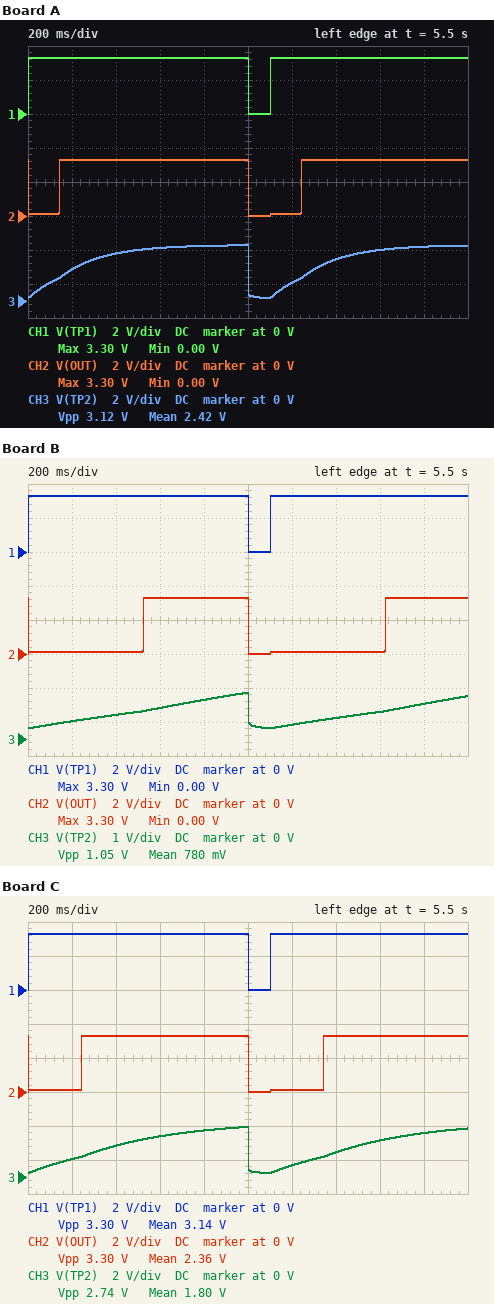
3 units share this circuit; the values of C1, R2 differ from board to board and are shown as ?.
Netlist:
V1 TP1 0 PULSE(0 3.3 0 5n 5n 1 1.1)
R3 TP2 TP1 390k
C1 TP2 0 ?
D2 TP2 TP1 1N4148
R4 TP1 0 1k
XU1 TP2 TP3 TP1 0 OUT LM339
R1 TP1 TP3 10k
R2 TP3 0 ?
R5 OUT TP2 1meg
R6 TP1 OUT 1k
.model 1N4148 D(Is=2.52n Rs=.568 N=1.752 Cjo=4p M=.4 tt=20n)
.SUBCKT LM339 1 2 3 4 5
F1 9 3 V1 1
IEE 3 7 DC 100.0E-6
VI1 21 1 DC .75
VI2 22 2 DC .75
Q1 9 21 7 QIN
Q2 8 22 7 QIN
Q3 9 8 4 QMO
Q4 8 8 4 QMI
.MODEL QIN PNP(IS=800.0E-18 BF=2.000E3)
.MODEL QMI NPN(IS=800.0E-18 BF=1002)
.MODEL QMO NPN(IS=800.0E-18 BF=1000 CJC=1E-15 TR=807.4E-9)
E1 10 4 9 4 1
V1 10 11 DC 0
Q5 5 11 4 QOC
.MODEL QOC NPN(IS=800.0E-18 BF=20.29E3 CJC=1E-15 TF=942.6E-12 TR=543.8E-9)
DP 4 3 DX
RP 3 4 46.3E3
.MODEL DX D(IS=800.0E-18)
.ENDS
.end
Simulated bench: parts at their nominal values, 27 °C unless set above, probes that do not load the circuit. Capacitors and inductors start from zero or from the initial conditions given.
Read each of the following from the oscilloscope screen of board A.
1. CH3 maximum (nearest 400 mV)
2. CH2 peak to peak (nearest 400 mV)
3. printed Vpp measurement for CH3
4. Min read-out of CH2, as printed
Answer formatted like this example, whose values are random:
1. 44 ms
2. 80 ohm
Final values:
1. 3.2 V
2. 3.2 V
3. 3.12 V
4. 0.00 V
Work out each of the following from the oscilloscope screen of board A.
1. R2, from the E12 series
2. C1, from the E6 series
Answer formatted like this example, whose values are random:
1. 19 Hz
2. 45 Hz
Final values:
1. 6.8 kΩ
2. 680 nF
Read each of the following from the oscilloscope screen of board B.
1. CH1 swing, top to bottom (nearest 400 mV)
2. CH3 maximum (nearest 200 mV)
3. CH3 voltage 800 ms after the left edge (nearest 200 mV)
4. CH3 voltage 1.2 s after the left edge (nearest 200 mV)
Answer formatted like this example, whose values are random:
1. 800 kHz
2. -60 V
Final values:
1. 3.2 V
2. 1.4 V
3. 1.2 V
4. 400 mV
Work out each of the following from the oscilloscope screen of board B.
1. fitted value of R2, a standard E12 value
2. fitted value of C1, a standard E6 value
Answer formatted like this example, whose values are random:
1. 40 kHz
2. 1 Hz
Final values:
1. 3.3 kΩ
2. 6.8 µF
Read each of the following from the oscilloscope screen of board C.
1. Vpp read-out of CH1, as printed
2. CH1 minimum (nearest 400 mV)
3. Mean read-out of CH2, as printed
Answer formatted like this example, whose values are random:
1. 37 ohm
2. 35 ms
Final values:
1. 3.30 V
2. 0 V
3. 2.36 V
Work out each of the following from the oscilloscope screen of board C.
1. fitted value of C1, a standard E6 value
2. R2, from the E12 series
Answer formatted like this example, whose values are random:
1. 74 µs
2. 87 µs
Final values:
1. 1.5 µF
2. 5.6 kΩ
